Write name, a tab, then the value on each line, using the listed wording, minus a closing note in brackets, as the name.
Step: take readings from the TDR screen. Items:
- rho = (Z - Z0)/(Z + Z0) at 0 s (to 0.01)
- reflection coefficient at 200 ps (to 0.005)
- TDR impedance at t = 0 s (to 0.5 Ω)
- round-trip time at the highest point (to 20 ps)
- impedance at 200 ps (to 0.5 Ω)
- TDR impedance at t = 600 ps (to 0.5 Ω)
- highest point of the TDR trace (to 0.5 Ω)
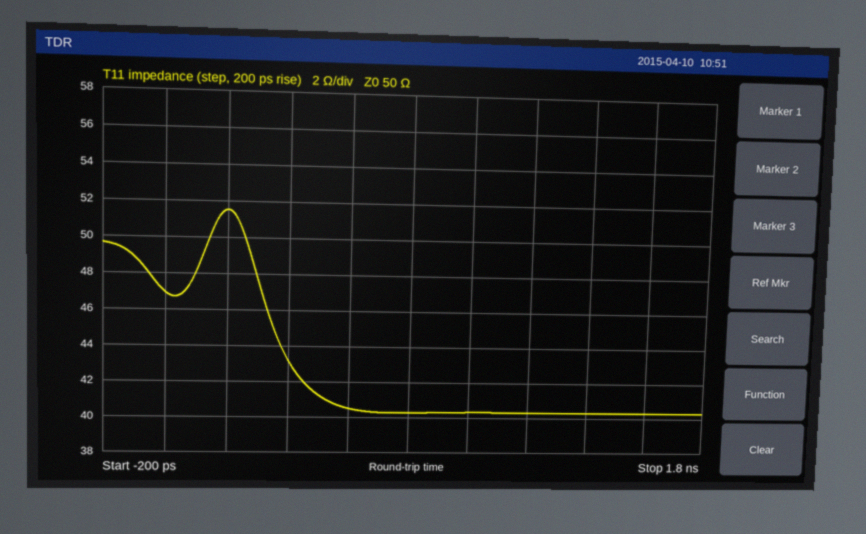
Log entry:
rho = (Z - Z0)/(Z + Z0) at 0 s	-0.03
reflection coefficient at 200 ps	+0.015
TDR impedance at t = 0 s	47.0 Ω
round-trip time at the highest point	200 ps
impedance at 200 ps	51.5 Ω
TDR impedance at t = 600 ps	40.5 Ω
highest point of the TDR trace	51.5 Ω
